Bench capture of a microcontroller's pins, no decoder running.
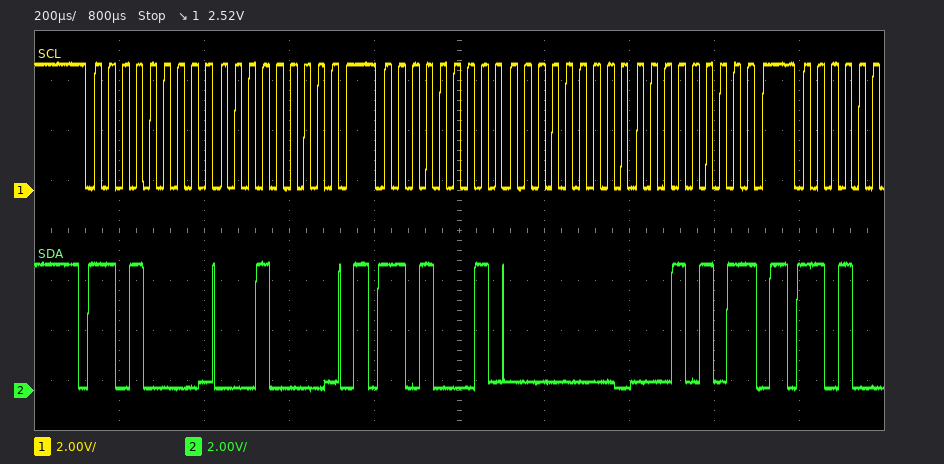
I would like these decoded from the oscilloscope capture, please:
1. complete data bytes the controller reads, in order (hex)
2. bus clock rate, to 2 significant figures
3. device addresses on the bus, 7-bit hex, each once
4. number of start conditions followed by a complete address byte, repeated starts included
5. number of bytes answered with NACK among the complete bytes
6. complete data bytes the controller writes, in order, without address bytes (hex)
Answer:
00 15
31 kHz
0x68
2
1
10
